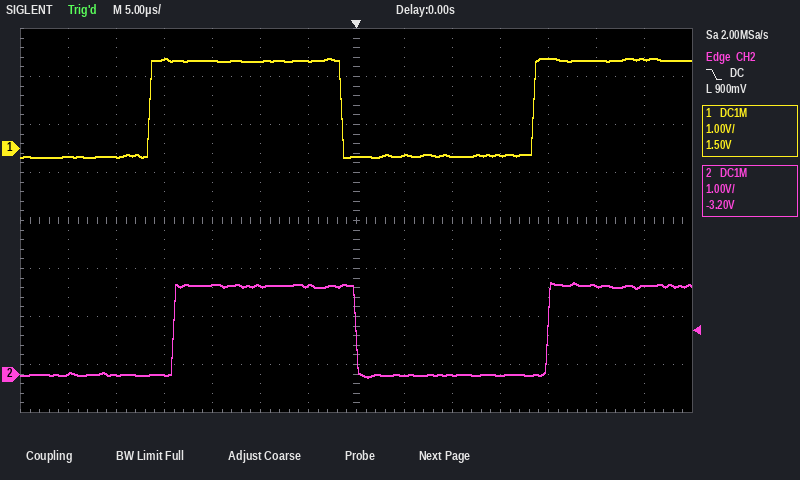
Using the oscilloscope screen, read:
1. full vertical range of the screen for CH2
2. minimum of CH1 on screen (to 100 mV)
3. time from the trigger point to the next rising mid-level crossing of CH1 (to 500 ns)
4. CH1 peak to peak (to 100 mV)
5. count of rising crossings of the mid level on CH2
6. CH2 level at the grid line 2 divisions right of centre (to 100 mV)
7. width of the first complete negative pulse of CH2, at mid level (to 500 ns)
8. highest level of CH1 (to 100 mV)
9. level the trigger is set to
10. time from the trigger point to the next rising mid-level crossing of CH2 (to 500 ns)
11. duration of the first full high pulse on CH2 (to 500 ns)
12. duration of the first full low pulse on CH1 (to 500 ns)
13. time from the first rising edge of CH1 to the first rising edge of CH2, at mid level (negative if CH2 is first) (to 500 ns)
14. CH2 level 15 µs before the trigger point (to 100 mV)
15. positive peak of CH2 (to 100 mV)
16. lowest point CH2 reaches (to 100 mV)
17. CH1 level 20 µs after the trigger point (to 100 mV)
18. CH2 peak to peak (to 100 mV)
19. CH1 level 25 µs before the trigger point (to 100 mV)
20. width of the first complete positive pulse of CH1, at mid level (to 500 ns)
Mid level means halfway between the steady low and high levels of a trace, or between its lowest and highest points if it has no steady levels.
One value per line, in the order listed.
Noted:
8 V
-200 mV
18.5 µs
2.1 V
2
0.0 V
20.0 µs
1.9 V
900 mV
20.0 µs
19.0 µs
20.0 µs
+2.5 µs
1.9 V
1.9 V
-100 mV
1.9 V
2.0 V
-200 mV
20.0 µs
